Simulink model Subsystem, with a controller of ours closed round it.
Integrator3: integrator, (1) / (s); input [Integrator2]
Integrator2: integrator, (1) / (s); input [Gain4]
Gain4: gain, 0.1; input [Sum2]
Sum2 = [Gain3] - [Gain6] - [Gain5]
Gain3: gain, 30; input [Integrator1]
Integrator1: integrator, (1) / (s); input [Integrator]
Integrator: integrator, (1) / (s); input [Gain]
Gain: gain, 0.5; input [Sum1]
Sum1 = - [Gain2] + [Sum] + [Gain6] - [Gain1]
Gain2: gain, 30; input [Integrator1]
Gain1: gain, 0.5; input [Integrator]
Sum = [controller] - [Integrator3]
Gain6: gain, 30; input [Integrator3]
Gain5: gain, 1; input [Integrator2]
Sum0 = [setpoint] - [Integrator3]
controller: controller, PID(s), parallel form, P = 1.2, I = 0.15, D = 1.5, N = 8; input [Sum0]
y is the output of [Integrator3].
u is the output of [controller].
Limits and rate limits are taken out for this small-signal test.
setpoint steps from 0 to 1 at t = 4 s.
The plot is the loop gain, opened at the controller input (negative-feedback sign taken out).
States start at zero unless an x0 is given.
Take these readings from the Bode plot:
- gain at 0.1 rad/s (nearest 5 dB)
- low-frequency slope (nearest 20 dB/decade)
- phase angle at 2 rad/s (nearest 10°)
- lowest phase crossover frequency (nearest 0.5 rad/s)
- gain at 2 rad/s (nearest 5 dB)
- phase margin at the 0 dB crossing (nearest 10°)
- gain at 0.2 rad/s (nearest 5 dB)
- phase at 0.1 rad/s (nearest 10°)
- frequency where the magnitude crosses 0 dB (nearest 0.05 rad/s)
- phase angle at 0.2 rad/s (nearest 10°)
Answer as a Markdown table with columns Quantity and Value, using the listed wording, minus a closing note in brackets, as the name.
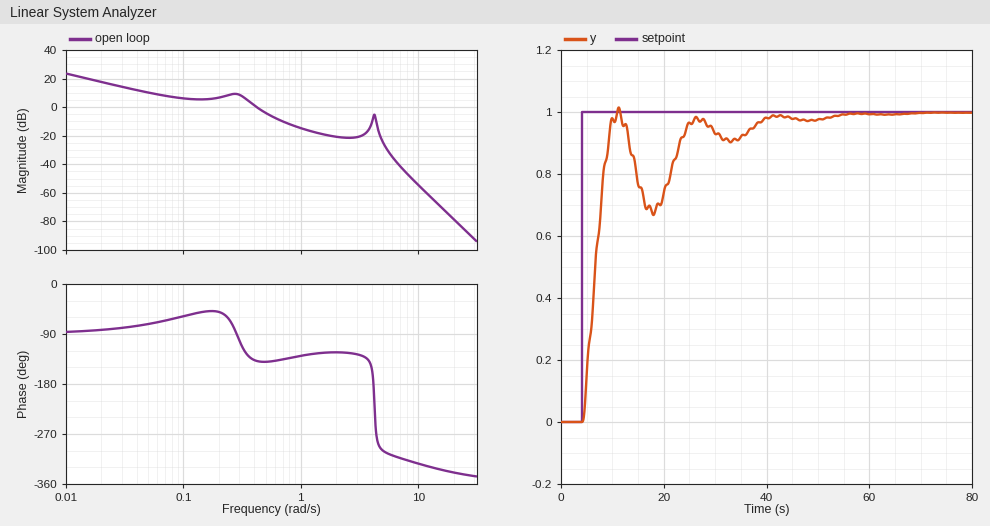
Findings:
| Quantity | Value |
|---|---|
| gain at 0.1 rad/s | 5 dB |
| low-frequency slope | -20 dB/decade |
| phase angle at 2 rad/s | -120° |
| lowest phase crossover frequency | 4.0 rad/s |
| gain at 2 rad/s | -20 dB |
| phase margin at the 0 dB crossing | 40° |
| gain at 0.2 rad/s | 5 dB |
| phase at 0.1 rad/s | -60° |
| frequency where the magnitude crosses 0 dB | 0.40 rad/s |
| phase angle at 0.2 rad/s | -50° |
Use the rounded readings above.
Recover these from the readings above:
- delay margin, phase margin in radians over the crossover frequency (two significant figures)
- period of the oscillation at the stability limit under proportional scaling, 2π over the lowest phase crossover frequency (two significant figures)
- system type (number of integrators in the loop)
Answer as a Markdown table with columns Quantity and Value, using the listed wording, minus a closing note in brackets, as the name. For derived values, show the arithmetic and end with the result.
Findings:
| Quantity | Value |
|---|---|
| delay margin, phase margin in radians over the crossover frequency | 40 × π / 180 / 0.4 = 1.7 s |
| period of the oscillation at the stability limit under proportional scaling, 2π over the lowest phase crossover frequency | 2π / 4 = 1.6 s |
| system type | 1 |
